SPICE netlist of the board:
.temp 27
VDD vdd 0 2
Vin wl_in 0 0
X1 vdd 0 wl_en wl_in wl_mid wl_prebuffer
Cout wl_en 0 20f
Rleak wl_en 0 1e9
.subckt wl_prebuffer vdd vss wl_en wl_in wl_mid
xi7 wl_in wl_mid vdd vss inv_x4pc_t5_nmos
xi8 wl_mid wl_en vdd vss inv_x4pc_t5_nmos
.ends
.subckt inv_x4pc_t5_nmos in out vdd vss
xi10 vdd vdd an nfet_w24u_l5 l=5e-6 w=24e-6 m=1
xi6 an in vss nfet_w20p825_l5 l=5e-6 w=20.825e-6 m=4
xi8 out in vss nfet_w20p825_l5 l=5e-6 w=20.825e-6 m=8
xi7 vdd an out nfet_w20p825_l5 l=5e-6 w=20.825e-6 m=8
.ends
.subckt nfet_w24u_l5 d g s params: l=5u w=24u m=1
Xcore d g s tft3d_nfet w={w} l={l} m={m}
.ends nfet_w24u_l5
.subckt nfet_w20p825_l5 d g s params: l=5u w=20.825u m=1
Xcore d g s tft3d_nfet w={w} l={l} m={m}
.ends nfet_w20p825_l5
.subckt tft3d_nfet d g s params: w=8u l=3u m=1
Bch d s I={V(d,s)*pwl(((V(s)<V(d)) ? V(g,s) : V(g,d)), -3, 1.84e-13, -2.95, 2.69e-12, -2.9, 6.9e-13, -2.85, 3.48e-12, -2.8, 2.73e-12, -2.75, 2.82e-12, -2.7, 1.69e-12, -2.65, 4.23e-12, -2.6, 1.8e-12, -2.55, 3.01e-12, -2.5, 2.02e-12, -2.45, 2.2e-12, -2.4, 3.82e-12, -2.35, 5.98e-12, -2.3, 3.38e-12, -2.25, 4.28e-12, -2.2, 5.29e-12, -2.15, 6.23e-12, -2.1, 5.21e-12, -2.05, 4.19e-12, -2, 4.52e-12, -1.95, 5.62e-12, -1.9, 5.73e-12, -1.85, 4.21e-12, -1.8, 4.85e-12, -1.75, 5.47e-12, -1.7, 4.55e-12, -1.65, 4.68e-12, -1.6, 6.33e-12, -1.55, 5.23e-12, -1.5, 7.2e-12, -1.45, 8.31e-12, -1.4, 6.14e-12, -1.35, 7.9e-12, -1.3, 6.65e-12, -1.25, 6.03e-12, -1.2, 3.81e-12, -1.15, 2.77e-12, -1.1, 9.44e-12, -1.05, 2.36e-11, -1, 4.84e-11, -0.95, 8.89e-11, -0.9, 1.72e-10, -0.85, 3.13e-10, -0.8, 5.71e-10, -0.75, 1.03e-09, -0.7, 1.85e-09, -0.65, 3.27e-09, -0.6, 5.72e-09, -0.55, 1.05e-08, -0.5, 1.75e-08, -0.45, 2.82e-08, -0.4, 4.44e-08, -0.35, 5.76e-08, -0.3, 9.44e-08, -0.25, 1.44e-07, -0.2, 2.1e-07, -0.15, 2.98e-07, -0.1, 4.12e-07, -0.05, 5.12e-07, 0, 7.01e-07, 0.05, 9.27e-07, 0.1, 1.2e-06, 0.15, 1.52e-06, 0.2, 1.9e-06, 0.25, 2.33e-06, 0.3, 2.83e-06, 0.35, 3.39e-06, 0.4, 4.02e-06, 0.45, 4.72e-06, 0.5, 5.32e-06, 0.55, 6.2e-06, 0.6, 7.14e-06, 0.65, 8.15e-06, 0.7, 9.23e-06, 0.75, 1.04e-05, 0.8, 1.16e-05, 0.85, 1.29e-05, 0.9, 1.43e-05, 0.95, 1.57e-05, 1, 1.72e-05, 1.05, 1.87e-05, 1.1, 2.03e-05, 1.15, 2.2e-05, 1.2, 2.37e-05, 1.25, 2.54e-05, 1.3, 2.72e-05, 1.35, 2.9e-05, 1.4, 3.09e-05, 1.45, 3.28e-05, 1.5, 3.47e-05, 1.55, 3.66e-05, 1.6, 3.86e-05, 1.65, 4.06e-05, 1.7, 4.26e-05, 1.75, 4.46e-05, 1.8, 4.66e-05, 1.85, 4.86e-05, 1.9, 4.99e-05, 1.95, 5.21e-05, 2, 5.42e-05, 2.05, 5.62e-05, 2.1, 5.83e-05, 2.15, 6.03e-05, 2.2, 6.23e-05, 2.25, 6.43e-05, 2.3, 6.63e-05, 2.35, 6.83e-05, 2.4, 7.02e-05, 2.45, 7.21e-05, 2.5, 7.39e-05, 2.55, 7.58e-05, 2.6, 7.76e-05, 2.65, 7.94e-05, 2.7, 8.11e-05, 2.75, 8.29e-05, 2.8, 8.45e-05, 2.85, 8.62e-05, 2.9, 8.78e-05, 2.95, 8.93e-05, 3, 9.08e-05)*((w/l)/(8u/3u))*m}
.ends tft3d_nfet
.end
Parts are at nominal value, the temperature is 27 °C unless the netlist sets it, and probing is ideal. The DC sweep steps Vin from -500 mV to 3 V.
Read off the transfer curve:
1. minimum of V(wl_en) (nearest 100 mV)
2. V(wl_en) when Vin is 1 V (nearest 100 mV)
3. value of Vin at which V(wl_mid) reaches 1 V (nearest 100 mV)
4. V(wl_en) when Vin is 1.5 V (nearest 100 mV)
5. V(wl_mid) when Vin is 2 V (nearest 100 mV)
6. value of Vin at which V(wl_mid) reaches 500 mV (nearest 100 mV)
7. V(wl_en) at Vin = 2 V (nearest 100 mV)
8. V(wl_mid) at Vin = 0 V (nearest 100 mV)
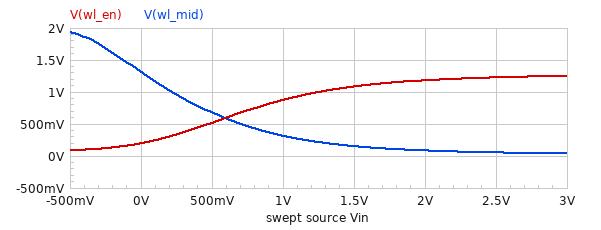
100 mV
900 mV
200 mV
1.1 V
100 mV
700 mV
1.2 V
1.3 V
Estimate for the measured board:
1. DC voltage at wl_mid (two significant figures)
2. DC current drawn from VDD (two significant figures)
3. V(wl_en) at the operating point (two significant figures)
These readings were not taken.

1.3 V
180 µA
200 mV
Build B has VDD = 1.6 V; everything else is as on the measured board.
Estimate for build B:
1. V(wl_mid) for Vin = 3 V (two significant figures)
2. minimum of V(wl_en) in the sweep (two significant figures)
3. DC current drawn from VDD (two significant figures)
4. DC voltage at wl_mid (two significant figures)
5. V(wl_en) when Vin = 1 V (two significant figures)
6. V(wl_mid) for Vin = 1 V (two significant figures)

24 mV
81 mV
100 µA
1.0 V
760 mV
190 mV
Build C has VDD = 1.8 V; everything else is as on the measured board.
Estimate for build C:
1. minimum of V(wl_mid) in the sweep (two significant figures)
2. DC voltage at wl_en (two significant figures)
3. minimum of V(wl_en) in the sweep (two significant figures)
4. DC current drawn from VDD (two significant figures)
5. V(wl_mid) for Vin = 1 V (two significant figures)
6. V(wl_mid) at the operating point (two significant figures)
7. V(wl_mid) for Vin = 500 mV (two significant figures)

32 mV
190 mV
86 mV
140 µA
250 mV
1.2 V
570 mV
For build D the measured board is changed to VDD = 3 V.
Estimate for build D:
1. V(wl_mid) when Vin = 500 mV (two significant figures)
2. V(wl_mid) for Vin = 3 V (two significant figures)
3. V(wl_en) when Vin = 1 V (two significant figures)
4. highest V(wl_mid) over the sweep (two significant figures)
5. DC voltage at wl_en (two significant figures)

1.3 V
140 mV
1.0 V
2.9 V
230 mV
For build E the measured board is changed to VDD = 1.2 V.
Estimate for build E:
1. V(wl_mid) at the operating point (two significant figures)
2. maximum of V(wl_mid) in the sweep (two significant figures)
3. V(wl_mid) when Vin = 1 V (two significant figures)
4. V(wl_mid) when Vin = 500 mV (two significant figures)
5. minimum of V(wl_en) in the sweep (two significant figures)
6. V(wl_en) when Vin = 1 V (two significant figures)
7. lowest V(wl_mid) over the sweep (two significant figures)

710 mV
1.2 V
98 mV
280 mV
73 mV
590 mV
13 mV
